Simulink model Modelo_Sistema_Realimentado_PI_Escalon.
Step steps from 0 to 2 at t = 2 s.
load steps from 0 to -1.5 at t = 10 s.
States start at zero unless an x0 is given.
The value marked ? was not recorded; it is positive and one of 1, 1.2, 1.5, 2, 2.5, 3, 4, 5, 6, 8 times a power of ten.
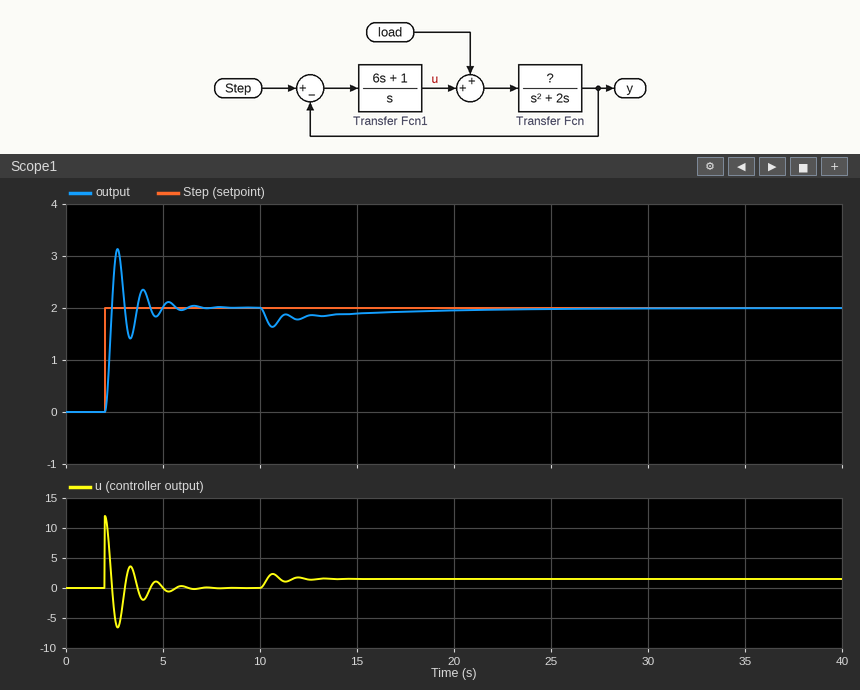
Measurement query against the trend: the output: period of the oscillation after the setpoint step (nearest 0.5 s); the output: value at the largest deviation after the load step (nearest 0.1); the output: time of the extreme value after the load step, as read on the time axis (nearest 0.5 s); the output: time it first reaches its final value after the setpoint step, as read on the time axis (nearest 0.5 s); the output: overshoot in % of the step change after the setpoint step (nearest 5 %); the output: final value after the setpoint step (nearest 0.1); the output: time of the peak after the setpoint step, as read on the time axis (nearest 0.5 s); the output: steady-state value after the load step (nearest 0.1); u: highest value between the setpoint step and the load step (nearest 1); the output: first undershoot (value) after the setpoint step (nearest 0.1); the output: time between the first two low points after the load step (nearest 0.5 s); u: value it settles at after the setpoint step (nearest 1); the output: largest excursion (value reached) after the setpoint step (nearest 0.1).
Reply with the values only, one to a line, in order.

1.5 s
1.6
10.5 s
2.5 s
55 %
2.0
2.5 s
2.0
12
1.4
1.5 s
0
3.1
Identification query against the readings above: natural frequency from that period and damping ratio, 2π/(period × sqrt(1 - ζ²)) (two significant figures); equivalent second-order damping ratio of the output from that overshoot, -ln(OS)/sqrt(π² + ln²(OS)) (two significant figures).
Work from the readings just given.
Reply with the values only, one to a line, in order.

4.3 rad/s
0.19
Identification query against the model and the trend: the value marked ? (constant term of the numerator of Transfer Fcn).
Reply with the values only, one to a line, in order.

4
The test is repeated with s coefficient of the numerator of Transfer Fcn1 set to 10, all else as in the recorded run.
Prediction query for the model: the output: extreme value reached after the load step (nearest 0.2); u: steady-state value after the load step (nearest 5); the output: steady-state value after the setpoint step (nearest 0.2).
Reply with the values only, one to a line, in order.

1.8
0
2.0
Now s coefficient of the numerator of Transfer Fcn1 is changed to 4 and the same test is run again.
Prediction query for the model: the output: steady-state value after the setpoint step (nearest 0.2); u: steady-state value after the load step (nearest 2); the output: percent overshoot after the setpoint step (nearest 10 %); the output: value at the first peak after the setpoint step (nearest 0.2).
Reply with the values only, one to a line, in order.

2.0
2
50 %
3.0
